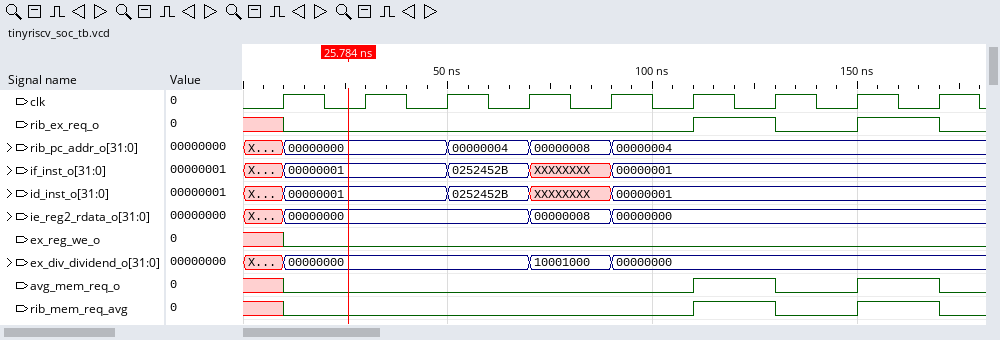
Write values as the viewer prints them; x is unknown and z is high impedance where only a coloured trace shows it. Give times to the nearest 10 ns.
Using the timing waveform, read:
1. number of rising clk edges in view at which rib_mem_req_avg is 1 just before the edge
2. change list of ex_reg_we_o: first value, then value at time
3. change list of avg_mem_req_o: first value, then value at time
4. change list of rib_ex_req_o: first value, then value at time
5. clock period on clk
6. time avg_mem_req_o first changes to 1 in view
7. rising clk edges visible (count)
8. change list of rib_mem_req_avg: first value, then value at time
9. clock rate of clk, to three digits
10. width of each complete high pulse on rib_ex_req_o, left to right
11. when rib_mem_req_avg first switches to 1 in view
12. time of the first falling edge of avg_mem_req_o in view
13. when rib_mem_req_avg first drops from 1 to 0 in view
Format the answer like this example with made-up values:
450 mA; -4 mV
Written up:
2; x, 0 at 10 ns; x, 0 at 10 ns, 1 at 110 ns, 0 at 130 ns, 1 at 150 ns, 0 at 170 ns; x, 0 at 10 ns, 1 at 110 ns, 0 at 130 ns, 1 at 150 ns, 0 at 170 ns; 20 ns; 110 ns; 9; x, 0 at 10 ns, 1 at 110 ns, 0 at 130 ns, 1 at 150 ns, 0 at 170 ns; 50.0 MHz; 20 ns, 20 ns; 110 ns; 130 ns; 130 ns
